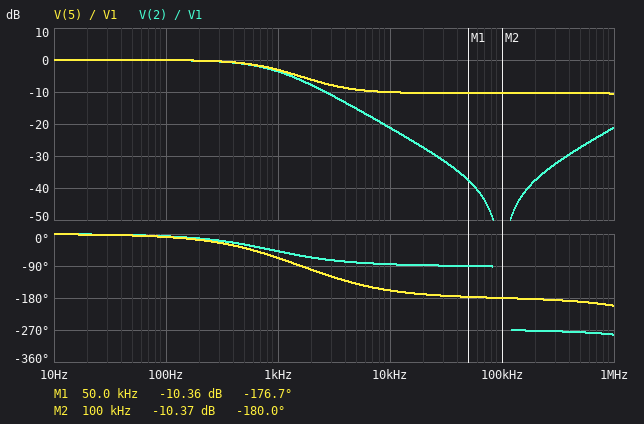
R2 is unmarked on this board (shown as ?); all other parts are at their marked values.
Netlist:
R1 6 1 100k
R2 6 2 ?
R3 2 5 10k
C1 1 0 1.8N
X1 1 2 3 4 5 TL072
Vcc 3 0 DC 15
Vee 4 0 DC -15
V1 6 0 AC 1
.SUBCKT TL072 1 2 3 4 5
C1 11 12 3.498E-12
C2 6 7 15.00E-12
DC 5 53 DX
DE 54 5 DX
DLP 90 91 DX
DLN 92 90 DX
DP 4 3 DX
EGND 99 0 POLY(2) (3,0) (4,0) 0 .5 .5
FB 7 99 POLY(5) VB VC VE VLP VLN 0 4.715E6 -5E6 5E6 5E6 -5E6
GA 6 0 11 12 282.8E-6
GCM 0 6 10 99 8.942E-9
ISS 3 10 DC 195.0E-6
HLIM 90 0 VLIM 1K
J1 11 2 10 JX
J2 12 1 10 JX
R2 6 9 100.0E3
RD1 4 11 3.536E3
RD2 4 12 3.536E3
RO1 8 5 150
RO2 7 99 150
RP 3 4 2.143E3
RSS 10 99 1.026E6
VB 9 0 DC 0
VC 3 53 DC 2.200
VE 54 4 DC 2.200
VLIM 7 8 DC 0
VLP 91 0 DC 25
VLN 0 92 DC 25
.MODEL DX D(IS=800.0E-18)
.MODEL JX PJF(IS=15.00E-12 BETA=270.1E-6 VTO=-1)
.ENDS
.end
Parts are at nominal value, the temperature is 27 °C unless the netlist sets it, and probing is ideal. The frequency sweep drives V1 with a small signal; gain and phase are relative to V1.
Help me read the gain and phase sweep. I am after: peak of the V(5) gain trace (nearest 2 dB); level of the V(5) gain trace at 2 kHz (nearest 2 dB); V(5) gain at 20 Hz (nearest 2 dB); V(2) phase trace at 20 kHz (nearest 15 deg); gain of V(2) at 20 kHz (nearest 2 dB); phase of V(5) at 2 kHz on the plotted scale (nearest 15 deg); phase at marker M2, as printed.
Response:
0 dB
-6 dB
0 dB
-90 deg
-28 dB
-105 deg
-180.0 deg
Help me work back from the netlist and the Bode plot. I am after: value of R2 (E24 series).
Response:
33 kΩ
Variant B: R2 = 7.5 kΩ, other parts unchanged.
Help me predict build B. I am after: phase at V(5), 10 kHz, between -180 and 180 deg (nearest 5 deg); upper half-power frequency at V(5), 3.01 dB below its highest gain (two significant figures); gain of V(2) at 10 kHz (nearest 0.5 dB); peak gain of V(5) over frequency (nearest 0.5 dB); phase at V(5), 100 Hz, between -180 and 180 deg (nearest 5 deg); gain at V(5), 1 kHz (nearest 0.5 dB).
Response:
-170 deg
1.9 MHz
-21.5 dB
2.5 dB
-15 deg
1.5 dB
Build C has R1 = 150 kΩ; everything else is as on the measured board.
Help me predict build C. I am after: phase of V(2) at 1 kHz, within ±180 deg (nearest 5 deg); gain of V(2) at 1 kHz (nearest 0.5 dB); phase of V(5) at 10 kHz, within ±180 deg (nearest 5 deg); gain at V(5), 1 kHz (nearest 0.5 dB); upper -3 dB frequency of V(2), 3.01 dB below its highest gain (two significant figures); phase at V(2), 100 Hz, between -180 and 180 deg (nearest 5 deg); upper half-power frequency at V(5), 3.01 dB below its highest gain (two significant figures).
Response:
-60 deg
-6.0 dB
-165 deg
-5.0 dB
590 Hz
-10 deg
650 Hz
